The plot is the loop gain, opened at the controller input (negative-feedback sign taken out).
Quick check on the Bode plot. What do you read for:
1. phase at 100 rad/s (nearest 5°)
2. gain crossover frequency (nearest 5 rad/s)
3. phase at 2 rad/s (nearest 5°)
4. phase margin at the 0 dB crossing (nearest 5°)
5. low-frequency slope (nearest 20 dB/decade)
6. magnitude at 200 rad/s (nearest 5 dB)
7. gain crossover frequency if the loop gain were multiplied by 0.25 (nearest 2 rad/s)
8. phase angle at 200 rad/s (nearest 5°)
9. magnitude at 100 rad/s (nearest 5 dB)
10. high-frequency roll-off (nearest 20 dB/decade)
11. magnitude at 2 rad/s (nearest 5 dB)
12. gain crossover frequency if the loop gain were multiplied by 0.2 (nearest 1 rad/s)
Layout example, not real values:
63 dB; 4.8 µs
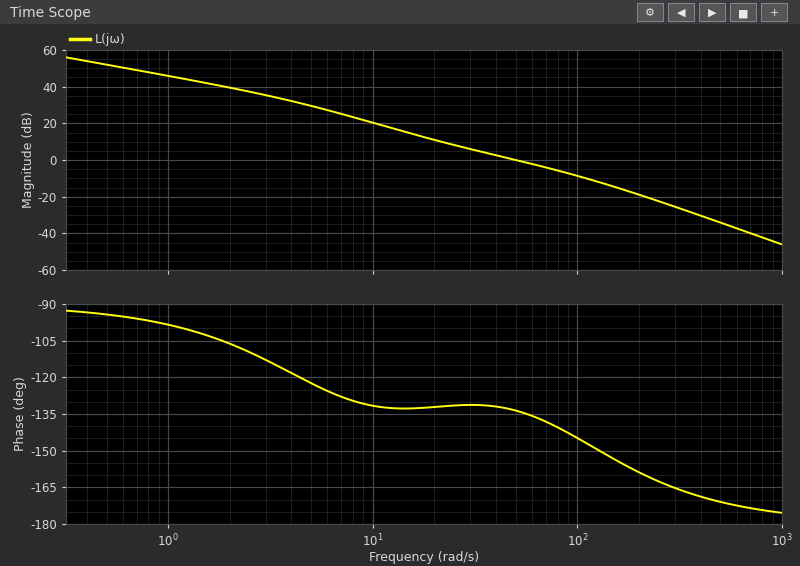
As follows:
-145°; 50 rad/s; -105°; 45°; -20 dB/decade; -20 dB; 18 rad/s; -160°; -10 dB; -40 dB/decade; 40 dB; 16 rad/s
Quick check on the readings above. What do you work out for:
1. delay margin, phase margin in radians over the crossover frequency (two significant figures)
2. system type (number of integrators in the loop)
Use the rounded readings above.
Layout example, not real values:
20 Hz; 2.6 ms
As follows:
0.016 s; 1
